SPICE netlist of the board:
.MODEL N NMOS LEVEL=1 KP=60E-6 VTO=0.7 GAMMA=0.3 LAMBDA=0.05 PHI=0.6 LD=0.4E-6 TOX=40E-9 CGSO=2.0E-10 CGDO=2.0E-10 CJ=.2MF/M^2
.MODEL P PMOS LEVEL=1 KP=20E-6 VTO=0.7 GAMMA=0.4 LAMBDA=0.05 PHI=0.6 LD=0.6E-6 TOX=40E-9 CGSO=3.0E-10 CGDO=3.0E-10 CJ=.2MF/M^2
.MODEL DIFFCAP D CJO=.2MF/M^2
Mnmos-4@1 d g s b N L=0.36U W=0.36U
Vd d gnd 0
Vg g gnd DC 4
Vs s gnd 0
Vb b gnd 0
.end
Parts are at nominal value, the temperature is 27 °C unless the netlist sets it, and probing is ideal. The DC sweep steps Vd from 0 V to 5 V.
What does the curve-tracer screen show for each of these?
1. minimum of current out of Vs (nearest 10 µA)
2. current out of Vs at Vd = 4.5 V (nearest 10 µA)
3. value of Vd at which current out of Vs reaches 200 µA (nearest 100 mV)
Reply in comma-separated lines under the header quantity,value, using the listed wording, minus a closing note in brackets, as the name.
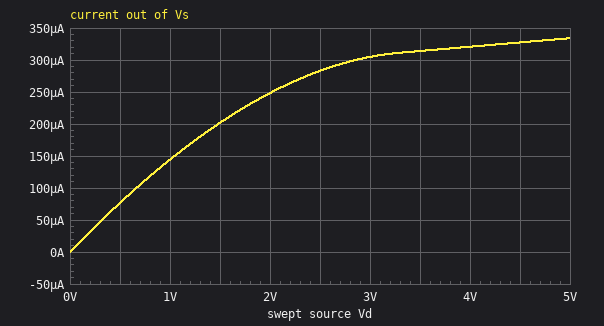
quantity,value
minimum of current out of Vs,0 A
current out of Vs at Vd = 4.5 V,330 µA
value of Vd at which current out of Vs reaches 200 µA,1.5 V
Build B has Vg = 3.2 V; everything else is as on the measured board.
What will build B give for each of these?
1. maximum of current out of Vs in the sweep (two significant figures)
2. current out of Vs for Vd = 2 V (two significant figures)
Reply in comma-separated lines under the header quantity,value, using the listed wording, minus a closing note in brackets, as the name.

quantity,value
maximum of current out of Vs in the sweep,190 µA
current out of Vs for Vd = 2 V,160 µA
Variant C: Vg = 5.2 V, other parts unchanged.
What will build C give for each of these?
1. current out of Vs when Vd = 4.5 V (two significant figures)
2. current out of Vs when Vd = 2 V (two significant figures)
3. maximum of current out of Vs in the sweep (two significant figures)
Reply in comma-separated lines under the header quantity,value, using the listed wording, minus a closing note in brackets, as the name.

quantity,value
current out of Vs when Vd = 4.5 V,610 µA
current out of Vs when Vd = 2 V,380 µA
maximum of current out of Vs in the sweep,620 µA
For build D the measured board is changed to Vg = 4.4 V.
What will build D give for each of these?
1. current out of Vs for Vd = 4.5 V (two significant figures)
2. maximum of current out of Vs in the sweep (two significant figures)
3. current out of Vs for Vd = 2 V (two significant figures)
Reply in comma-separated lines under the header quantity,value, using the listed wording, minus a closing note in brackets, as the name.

quantity,value
current out of Vs for Vd = 4.5 V,410 µA
maximum of current out of Vs in the sweep,420 µA
current out of Vs for Vd = 2 V,290 µA
